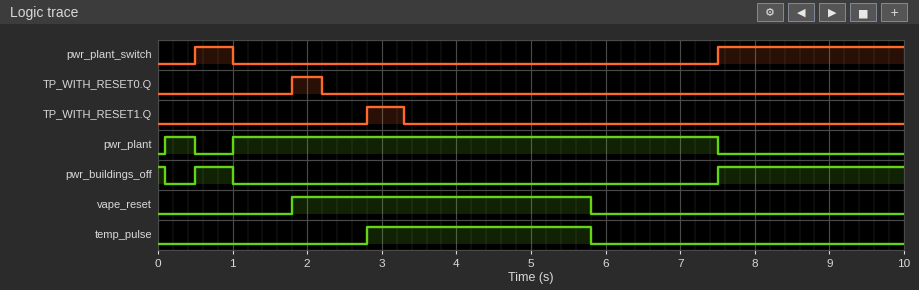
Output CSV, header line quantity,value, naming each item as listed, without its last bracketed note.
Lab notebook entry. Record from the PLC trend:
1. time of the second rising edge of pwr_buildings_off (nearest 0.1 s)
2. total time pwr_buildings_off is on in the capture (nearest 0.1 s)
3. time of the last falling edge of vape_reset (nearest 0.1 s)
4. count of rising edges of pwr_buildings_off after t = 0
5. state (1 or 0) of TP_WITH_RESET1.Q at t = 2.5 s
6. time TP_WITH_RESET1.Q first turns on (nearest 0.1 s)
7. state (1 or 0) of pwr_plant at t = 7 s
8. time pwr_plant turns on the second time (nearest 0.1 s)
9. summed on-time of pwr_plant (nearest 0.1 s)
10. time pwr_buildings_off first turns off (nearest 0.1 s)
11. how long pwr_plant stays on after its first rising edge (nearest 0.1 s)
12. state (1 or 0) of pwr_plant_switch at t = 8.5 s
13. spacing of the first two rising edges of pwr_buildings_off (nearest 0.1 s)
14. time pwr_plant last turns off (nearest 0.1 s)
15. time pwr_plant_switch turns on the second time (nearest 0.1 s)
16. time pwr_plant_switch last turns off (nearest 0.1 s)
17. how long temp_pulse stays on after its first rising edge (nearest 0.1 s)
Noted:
quantity,value
time of the second rising edge of pwr_buildings_off,7.5 s
total time pwr_buildings_off is on in the capture,3.1 s
time of the last falling edge of vape_reset,5.8 s
count of rising edges of pwr_buildings_off after t = 0,2
state (1 or 0) of TP_WITH_RESET1.Q at t = 2.5 s,0
time TP_WITH_RESET1.Q first turns on,2.8 s
state (1 or 0) of pwr_plant at t = 7 s,1
time pwr_plant turns on the second time,1.0 s
summed on-time of pwr_plant,6.9 s
time pwr_buildings_off first turns off,0.1 s
how long pwr_plant stays on after its first rising edge,0.4 s
state (1 or 0) of pwr_plant_switch at t = 8.5 s,1
spacing of the first two rising edges of pwr_buildings_off,7.0 s
time pwr_plant last turns off,7.5 s
time pwr_plant_switch turns on the second time,7.5 s
time pwr_plant_switch last turns off,1.0 s
how long temp_pulse stays on after its first rising edge,3.0 s
